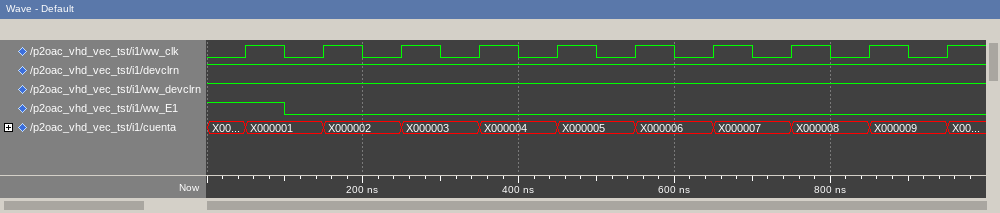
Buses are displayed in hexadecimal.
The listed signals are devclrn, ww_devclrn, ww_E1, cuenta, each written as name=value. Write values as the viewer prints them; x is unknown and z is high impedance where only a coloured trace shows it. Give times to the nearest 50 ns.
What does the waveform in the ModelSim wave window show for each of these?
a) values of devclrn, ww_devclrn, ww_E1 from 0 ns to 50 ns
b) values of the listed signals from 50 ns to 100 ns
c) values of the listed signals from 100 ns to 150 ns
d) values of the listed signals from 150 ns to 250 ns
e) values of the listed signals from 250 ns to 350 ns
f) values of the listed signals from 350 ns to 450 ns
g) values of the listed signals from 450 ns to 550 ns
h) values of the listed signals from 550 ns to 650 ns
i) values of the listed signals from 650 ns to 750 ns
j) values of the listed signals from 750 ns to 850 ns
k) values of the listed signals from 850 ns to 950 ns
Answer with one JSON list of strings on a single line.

["devclrn=1, ww_devclrn=1, ww_E1=1", "devclrn=1, ww_devclrn=1, ww_E1=1, cuenta=X000001", "devclrn=1, ww_devclrn=1, ww_E1=0, cuenta=X000001", "devclrn=1, ww_devclrn=1, ww_E1=0, cuenta=X000002", "devclrn=1, ww_devclrn=1, ww_E1=0, cuenta=X000003", "devclrn=1, ww_devclrn=1, ww_E1=0, cuenta=X000004", "devclrn=1, ww_devclrn=1, ww_E1=0, cuenta=X000005", "devclrn=1, ww_devclrn=1, ww_E1=0, cuenta=X000006", "devclrn=1, ww_devclrn=1, ww_E1=0, cuenta=X000007", "devclrn=1, ww_devclrn=1, ww_E1=0, cuenta=X000008", "devclrn=1, ww_devclrn=1, ww_E1=0, cuenta=X000009"]
